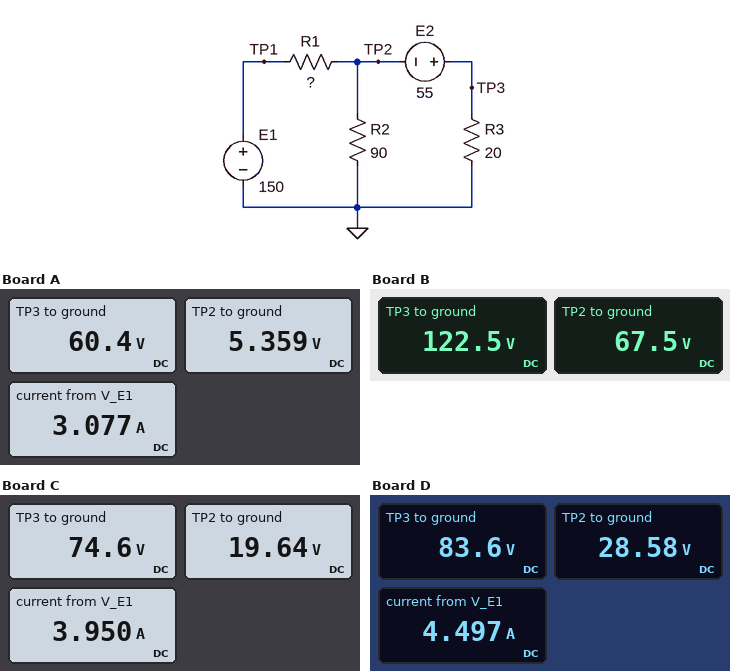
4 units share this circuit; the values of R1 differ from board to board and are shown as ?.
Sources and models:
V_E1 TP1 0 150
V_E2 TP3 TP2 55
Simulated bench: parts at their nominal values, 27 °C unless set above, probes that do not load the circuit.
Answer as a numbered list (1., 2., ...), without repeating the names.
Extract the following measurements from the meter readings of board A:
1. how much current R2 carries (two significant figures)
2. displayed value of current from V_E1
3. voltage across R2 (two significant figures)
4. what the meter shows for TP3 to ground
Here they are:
1. 60 mA
2. 3.077 A
3. 5.4 V
4. 60.4 V
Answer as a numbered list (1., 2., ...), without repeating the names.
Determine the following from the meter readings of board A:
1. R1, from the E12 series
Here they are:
1. 47 Ω
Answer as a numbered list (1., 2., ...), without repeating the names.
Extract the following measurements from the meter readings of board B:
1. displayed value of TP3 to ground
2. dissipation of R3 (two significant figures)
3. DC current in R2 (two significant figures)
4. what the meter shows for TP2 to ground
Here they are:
1. 122.5 V
2. 750 W
3. 750 mA
4. 67.5 V
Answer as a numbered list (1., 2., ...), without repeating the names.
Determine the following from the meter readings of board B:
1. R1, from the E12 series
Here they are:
1. 12 Ω
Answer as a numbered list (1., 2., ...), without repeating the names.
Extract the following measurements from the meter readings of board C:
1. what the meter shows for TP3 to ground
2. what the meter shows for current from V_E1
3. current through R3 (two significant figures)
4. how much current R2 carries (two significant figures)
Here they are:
1. 74.6 V
2. 3.950 A
3. 3.7 A
4. 220 mA
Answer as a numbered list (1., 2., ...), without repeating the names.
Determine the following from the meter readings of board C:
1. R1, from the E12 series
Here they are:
1. 33 Ω
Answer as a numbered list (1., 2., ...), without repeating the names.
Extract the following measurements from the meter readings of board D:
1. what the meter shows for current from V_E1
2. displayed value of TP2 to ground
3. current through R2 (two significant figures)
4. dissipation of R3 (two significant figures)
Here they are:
1. 4.497 A
2. 28.58 V
3. 320 mA
4. 350 W
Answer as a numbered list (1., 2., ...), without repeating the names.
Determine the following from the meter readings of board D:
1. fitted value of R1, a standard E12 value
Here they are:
1. 27 Ω
